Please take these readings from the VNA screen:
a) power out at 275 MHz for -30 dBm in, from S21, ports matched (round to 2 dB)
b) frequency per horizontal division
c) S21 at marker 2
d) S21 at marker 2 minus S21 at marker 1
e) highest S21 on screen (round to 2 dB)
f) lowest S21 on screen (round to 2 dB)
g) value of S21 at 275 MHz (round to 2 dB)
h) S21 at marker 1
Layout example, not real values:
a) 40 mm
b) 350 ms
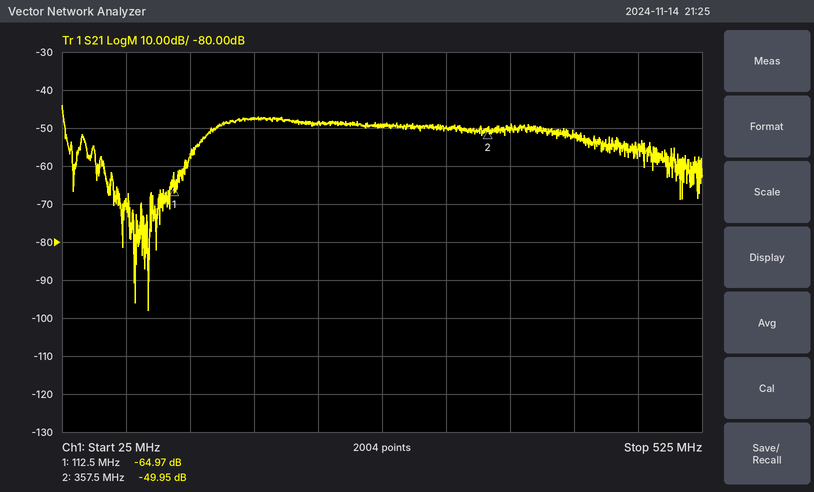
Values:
a) -80 dBm
b) 50 MHz
c) -49.95 dB
d) 15.02 dB
e) -44 dB
f) -98 dB
g) -50 dB
h) -64.97 dB
